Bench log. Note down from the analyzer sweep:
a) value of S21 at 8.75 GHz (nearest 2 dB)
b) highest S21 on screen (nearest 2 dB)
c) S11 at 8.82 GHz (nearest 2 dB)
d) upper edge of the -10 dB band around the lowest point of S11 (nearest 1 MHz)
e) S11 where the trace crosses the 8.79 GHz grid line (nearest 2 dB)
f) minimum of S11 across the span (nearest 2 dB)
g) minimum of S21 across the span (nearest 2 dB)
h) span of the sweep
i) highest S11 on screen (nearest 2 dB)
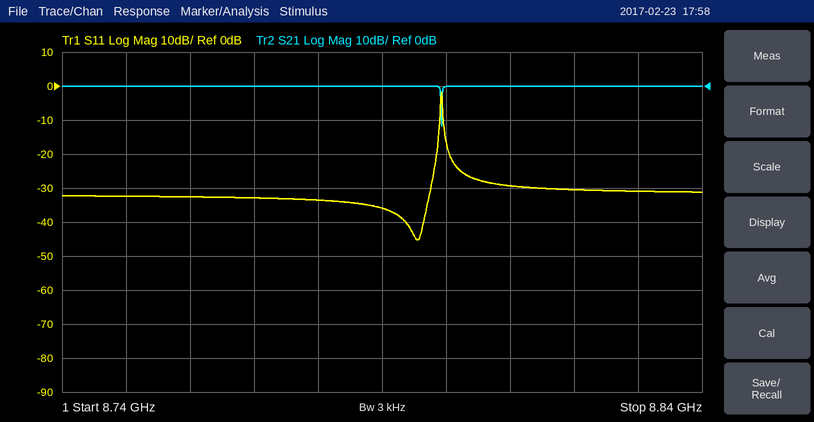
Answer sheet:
0 dB
0 dB
-30 dB
8.799 GHz
-36 dB
-46 dB
-12 dB
100 MHz
-2 dB
